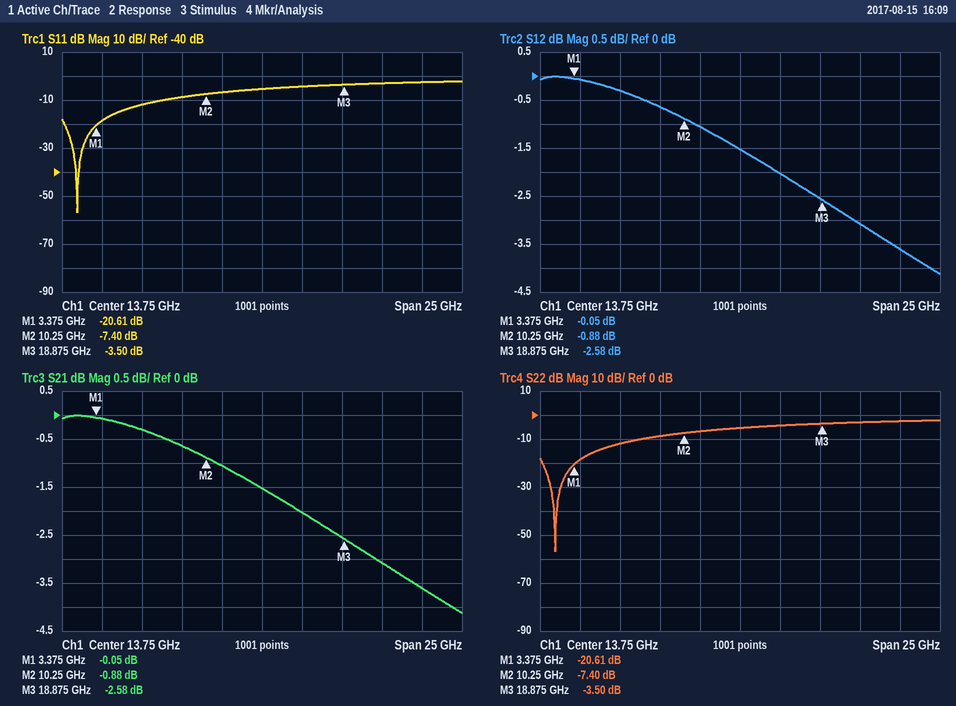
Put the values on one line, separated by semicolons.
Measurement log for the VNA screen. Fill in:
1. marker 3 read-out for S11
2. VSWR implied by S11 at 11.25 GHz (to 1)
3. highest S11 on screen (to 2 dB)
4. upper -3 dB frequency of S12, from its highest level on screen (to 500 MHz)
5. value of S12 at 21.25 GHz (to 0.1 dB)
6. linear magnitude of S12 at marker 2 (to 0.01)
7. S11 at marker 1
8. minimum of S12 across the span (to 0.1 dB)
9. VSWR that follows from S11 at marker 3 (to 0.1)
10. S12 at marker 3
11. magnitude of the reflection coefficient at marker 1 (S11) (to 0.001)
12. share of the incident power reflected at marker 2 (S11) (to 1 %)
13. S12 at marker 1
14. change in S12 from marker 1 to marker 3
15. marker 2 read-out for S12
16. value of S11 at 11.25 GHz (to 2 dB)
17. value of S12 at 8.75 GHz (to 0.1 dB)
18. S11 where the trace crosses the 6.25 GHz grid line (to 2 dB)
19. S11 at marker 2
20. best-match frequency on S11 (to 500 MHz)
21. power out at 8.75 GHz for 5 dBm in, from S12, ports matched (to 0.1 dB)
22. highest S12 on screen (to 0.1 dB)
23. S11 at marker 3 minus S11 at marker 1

-3.50 dB; 3; -2 dB; 21.0 GHz; -3.1 dB; 0.90; -20.61 dB; -4.1 dB; 5.0; -2.58 dB; 0.093; 18 %; -0.05 dB; -2.53 dB; -0.88 dB; -6 dB; -0.6 dB; -12 dB; -7.40 dB; 2.0 GHz; 4.4 dBm; 0.0 dB; 17.11 dB
